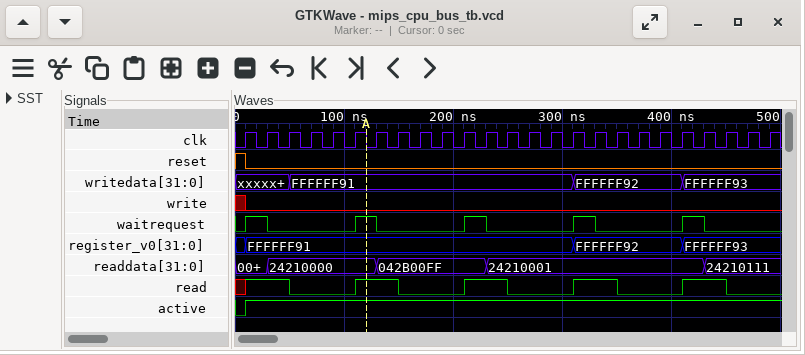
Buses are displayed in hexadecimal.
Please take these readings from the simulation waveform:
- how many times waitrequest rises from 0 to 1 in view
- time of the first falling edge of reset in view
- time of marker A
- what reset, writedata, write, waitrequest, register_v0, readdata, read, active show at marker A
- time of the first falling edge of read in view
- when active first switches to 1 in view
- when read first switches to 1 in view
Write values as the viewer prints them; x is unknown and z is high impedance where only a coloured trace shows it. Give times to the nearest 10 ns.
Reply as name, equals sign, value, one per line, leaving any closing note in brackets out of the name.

how many times waitrequest rises from 0 to 1 in view = 5
time of the first falling edge of reset in view = 10 ns
time of marker A = 120 ns
what reset, writedata, write, waitrequest, register_v0, readdata, read, active show at marker A = reset=0, writedata=FFFFFF91, write=0, waitrequest=1, register_v0=FFFFFF91, readdata=24210000, read=1, active=1
time of the first falling edge of read in view = 50 ns
when active first switches to 1 in view = 10 ns
when read first switches to 1 in view = 10 ns
